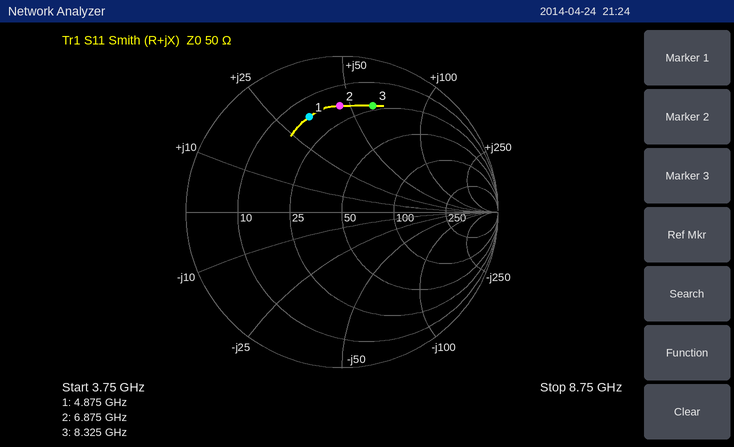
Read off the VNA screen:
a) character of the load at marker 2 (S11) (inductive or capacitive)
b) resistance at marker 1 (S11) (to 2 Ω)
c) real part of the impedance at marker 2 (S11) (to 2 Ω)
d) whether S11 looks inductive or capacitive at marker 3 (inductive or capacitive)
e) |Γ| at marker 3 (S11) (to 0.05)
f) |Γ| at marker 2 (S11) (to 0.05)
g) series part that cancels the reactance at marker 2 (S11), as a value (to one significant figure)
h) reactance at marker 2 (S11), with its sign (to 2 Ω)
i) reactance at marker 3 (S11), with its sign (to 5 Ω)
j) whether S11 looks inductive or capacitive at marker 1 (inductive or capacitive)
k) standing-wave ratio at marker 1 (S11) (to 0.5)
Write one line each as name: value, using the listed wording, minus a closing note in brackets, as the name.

character of the load at marker 2 (S11): inductive
resistance at marker 1 (S11): 16 Ω
real part of the impedance at marker 2 (S11): 18 Ω
whether S11 looks inductive or capacitive at marker 3: inductive
|Γ| at marker 3 (S11): 0.70
|Γ| at marker 2 (S11): 0.70
series part that cancels the reactance at marker 2 (S11), as a value: 500 fF
reactance at marker 2 (S11), with its sign: +46 Ω
reactance at marker 3 (S11), with its sign: +60 Ω
whether S11 looks inductive or capacitive at marker 1: inductive
standing-wave ratio at marker 1 (S11): 4.5
